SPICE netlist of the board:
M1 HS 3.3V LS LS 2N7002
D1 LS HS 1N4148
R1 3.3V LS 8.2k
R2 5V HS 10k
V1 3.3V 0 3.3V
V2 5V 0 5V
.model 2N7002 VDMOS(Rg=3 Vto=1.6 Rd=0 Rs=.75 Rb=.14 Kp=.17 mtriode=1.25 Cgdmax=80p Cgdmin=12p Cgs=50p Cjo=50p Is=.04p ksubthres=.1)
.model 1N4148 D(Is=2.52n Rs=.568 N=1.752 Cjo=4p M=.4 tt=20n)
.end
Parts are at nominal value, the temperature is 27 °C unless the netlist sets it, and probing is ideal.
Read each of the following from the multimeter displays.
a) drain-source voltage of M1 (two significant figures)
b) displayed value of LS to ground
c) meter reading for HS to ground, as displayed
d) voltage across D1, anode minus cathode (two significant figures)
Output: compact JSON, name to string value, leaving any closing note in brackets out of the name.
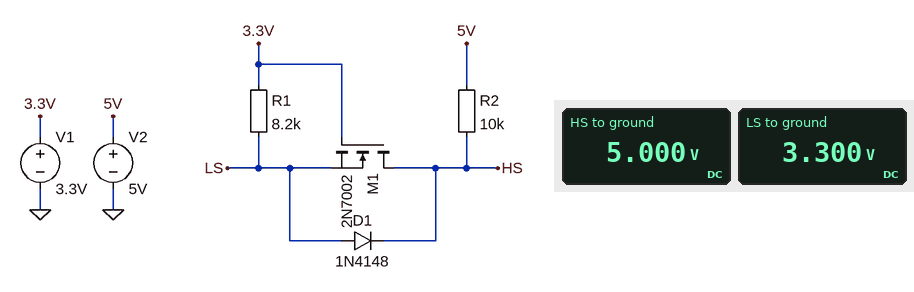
{"drain-source voltage of M1": "1.7 V", "displayed value of LS to ground": "3.300 V", "meter reading for HS to ground, as displayed": "5.000 V", "voltage across D1, anode minus cathode": "-1.7 V"}
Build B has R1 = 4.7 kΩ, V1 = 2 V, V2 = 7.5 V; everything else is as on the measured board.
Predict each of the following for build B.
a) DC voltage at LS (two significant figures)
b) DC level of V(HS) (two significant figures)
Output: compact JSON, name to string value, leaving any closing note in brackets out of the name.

{"DC voltage at LS": "2.0 V", "DC level of V(HS)": "7.5 V"}
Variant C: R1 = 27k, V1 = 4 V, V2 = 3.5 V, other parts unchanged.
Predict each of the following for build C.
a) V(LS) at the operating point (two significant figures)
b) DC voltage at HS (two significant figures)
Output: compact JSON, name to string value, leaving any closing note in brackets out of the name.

{"V(LS) at the operating point": "3.9 V", "DC voltage at HS": "3.5 V"}
